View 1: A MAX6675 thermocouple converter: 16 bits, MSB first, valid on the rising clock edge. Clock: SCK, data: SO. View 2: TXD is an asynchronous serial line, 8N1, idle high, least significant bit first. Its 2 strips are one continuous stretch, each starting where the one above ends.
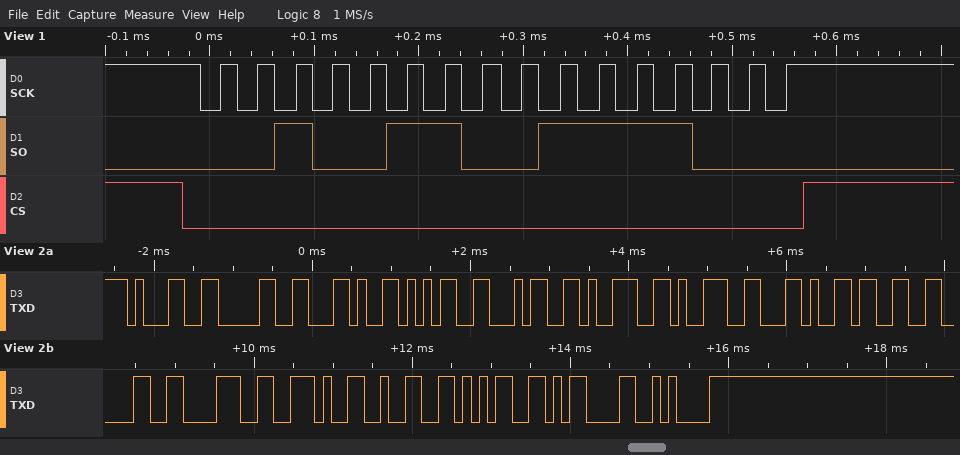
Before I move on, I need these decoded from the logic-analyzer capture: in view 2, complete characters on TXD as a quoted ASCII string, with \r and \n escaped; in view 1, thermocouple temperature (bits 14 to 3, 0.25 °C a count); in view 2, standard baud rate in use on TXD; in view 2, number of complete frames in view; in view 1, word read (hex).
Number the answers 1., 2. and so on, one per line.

1. "10,5499,308.25\r\n"
2. 307.75 °C
3. 9600 baud
4. 16
5. 0x2678
